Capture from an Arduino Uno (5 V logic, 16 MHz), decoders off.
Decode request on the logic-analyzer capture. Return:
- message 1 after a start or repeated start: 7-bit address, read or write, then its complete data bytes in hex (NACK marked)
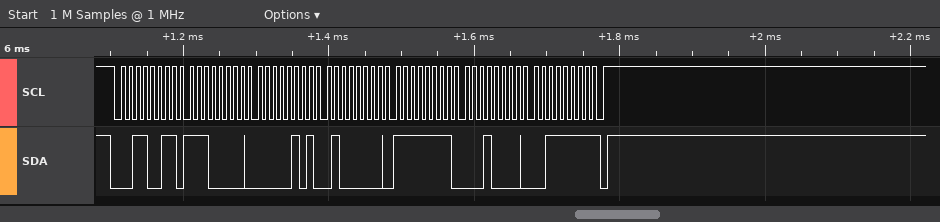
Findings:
0x19 read: E0 05 40 FF 10 3F NACK
